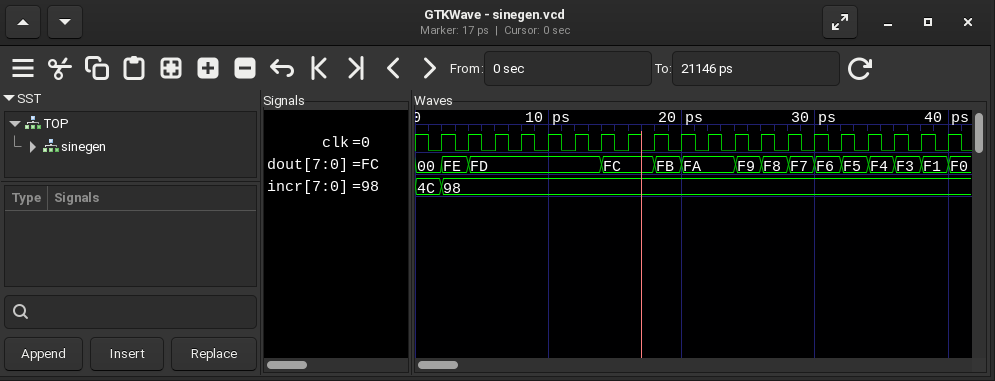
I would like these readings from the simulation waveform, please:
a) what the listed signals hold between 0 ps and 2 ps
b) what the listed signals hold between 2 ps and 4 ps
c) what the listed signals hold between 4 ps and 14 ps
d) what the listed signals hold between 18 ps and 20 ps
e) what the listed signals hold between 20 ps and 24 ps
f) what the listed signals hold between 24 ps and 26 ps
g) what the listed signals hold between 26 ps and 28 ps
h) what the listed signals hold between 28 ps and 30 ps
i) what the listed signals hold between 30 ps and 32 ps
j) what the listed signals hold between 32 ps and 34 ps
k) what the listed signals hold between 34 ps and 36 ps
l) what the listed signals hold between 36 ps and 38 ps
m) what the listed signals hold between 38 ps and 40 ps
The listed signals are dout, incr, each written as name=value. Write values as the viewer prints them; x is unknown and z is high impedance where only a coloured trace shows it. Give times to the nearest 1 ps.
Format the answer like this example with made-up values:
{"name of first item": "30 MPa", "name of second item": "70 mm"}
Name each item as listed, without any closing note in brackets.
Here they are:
{"what the listed signals hold between 0 ps and 2 ps": "dout=00, incr=4C", "what the listed signals hold between 2 ps and 4 ps": "dout=FE, incr=98", "what the listed signals hold between 4 ps and 14 ps": "dout=FD, incr=98", "what the listed signals hold between 18 ps and 20 ps": "dout=FB, incr=98", "what the listed signals hold between 20 ps and 24 ps": "dout=FA, incr=98", "what the listed signals hold between 24 ps and 26 ps": "dout=F9, incr=98", "what the listed signals hold between 26 ps and 28 ps": "dout=F8, incr=98", "what the listed signals hold between 28 ps and 30 ps": "dout=F7, incr=98", "what the listed signals hold between 30 ps and 32 ps": "dout=F6, incr=98", "what the listed signals hold between 32 ps and 34 ps": "dout=F5, incr=98", "what the listed signals hold between 34 ps and 36 ps": "dout=F4, incr=98", "what the listed signals hold between 36 ps and 38 ps": "dout=F3, incr=98", "what the listed signals hold between 38 ps and 40 ps": "dout=F1, incr=98"}
